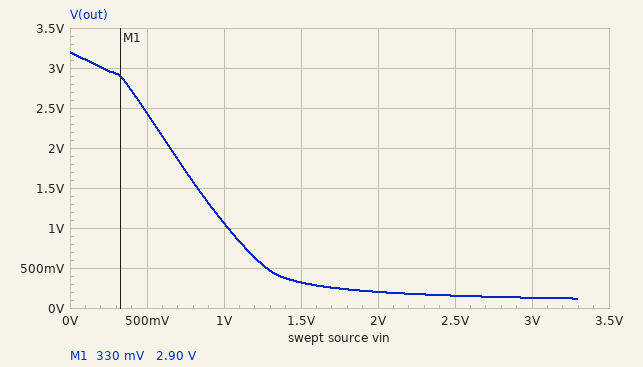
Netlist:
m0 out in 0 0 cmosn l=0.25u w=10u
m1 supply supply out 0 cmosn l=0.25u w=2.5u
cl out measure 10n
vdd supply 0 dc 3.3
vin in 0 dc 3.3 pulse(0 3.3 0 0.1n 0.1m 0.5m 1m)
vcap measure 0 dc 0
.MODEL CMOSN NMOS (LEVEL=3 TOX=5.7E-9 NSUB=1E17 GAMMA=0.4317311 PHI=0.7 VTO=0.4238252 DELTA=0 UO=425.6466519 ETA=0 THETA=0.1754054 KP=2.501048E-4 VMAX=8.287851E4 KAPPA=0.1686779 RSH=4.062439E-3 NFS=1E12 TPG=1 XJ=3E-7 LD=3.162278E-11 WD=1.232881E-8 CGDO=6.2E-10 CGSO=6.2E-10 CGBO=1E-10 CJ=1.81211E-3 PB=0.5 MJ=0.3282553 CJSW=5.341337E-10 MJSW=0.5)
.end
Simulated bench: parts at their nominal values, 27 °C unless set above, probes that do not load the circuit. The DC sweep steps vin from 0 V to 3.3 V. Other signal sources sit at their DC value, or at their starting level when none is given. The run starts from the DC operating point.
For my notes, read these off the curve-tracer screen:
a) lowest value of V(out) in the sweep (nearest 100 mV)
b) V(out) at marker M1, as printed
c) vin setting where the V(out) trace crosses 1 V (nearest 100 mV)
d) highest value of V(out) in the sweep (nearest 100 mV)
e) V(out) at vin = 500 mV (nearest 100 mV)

100 mV
2.90 V
1.0 V
3.2 V
2.4 V
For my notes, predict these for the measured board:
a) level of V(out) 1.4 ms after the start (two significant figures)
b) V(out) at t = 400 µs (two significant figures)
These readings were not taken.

120 mV
120 mV
